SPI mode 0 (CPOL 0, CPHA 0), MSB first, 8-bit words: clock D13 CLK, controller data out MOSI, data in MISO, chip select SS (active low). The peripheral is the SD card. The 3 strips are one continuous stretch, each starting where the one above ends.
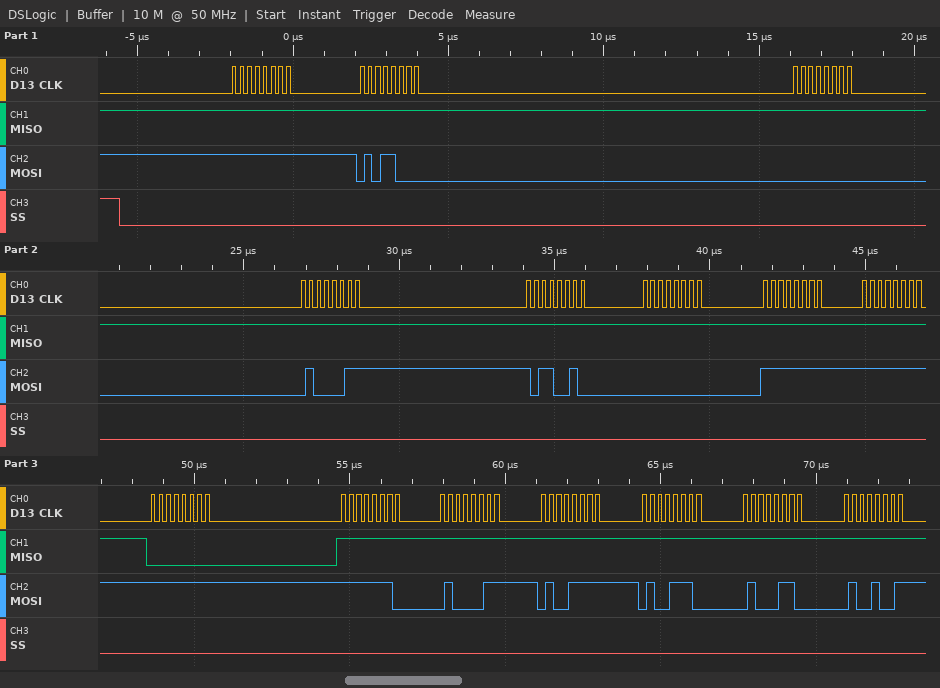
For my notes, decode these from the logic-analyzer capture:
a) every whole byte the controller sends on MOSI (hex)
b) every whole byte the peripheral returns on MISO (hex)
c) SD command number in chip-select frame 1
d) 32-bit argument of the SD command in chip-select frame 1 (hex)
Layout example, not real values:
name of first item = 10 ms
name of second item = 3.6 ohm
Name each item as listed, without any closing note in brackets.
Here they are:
every whole byte the controller sends on MOSI = FF 58 00 43 B2 00 FF FF FF FE 43 4F 4E 46 49
every whole byte the peripheral returns on MISO = FF FF FF FF FF FF FF FF 00 FF FF FF FF FF FF
SD command number in chip-select frame 1 = CMD24
32-bit argument of the SD command in chip-select frame 1 = 0x0043B200
